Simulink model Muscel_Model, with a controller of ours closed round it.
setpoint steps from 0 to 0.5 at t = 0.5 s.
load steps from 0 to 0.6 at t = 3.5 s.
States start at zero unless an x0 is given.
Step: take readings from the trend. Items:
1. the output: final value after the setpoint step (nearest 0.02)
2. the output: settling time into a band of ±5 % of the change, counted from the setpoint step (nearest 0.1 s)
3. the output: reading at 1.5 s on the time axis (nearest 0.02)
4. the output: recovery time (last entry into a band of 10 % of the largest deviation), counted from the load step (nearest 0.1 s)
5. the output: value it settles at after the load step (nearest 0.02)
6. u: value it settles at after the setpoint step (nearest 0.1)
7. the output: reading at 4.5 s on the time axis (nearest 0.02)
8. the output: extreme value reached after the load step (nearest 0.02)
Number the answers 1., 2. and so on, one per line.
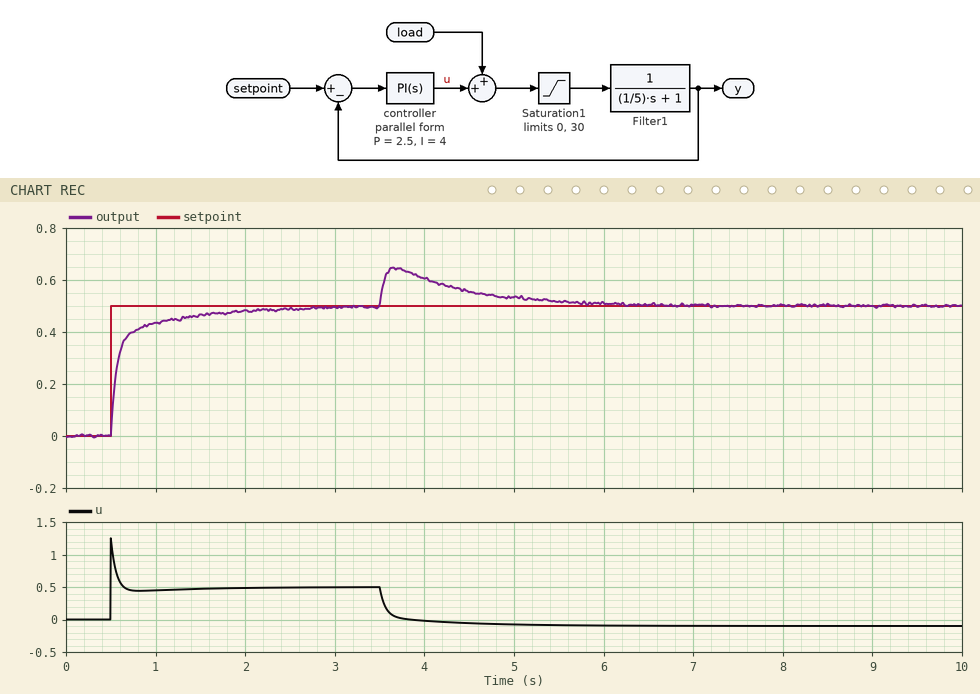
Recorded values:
1. 0.50
2. 1.3 s
3. 0.46
4. 2.1 s
5. 0.50
6. 0.5
7. 0.56
8. 0.64
